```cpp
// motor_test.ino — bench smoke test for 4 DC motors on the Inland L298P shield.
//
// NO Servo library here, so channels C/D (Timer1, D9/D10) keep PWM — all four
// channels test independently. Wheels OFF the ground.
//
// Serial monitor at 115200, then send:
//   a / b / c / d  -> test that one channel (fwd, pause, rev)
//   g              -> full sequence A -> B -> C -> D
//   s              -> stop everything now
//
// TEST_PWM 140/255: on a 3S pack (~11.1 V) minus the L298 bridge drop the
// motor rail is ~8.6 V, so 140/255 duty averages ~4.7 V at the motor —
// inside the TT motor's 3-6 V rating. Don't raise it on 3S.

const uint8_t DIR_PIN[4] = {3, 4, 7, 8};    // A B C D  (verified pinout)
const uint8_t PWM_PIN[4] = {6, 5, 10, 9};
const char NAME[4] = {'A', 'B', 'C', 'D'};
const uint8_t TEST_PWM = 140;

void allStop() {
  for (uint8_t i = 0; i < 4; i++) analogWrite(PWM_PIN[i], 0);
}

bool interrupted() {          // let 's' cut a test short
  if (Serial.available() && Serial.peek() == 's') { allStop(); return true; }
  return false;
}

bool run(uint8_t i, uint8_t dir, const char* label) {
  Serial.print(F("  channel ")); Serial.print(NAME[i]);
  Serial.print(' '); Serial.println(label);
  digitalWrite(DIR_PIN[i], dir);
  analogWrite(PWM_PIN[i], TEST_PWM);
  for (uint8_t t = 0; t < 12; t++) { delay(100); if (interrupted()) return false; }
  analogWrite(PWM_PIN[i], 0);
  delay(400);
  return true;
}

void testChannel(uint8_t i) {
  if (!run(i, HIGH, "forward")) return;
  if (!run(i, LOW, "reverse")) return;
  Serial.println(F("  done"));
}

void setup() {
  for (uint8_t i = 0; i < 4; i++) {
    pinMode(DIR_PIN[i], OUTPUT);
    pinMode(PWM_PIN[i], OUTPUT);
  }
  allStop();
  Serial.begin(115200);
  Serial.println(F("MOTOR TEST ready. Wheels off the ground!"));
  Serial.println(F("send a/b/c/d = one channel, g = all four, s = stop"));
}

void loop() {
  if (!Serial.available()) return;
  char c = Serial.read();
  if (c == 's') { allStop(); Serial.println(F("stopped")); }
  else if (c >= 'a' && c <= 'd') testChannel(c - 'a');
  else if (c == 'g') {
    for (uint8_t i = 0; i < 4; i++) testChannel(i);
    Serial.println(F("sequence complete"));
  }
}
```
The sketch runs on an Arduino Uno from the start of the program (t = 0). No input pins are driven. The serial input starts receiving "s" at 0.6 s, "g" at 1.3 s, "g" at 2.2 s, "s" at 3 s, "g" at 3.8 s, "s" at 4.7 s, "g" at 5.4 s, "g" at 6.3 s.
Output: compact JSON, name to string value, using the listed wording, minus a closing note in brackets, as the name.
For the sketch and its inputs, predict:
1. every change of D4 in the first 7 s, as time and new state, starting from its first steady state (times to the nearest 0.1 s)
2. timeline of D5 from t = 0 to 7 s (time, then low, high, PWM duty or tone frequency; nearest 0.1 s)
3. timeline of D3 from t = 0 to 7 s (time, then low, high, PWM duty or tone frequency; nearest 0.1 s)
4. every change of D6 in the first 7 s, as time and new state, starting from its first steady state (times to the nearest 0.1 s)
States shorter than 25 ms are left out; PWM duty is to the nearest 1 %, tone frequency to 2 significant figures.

{"every change of D4 in the first 7 s, as time and new state, starting from its first steady state": "0 s low; 4.5 s high; 6.1 s low", "timeline of D5 from t = 0 to 7 s": "0 s low; 4.5 s PWM 55 %; 5.7 s low; 6.1 s PWM 55 %", "timeline of D3 from t = 0 to 7 s": "0 s low; 1.3 s high; 2.9 s low", "every change of D6 in the first 7 s, as time and new state, starting from its first steady state": "0 s low; 1.3 s PWM 55 %; 2.5 s low; 2.9 s PWM 55 %; 4.1 s low"}
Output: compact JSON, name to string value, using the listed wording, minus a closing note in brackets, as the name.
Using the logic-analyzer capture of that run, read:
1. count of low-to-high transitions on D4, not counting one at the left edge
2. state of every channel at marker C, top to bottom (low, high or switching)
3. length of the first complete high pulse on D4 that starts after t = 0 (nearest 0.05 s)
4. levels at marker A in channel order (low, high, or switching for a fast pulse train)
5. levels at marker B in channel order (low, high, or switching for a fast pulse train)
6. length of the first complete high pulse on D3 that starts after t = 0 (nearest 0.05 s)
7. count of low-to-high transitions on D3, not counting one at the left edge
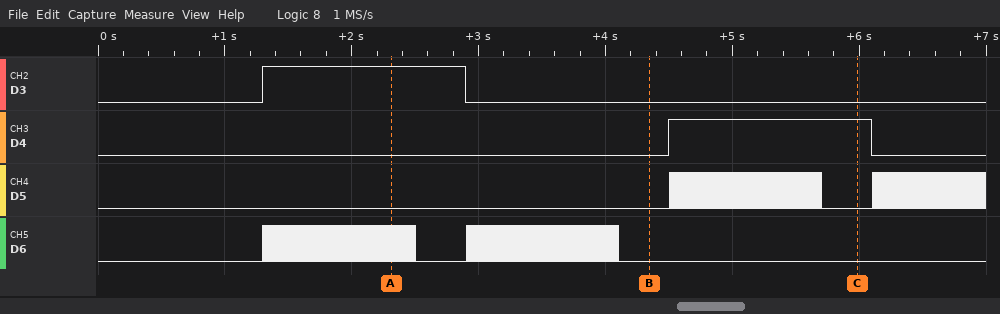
{"count of low-to-high transitions on D4, not counting one at the left edge": "1", "state of every channel at marker C, top to bottom": "D3 low, D4 high, D5 low, D6 low", "length of the first complete high pulse on D4 that starts after t = 0": "1.60 s", "levels at marker A in channel order": "D3 high, D4 low, D5 low, D6 switching", "levels at marker B in channel order": "D3 low, D4 low, D5 low, D6 low", "length of the first complete high pulse on D3 that starts after t = 0": "1.60 s", "count of low-to-high transitions on D3, not counting one at the left edge": "1"}
